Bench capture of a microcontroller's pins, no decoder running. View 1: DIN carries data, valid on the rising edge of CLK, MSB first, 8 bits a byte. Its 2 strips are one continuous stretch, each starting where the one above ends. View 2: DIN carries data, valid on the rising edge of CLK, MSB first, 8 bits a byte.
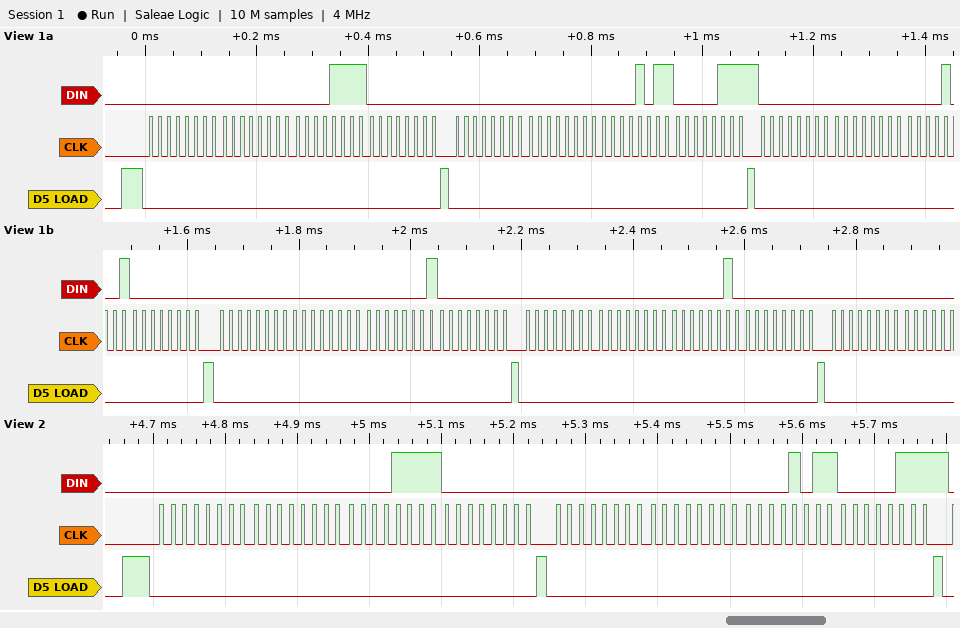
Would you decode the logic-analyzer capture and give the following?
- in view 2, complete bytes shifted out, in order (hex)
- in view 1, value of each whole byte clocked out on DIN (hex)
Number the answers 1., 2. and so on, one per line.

1. 00 00 0F 00 00 00 0B 07
2. 00 00 0F 00 00 00 0B 07 00 00 09 00 00 00 01 00 00 00 02 00 00
